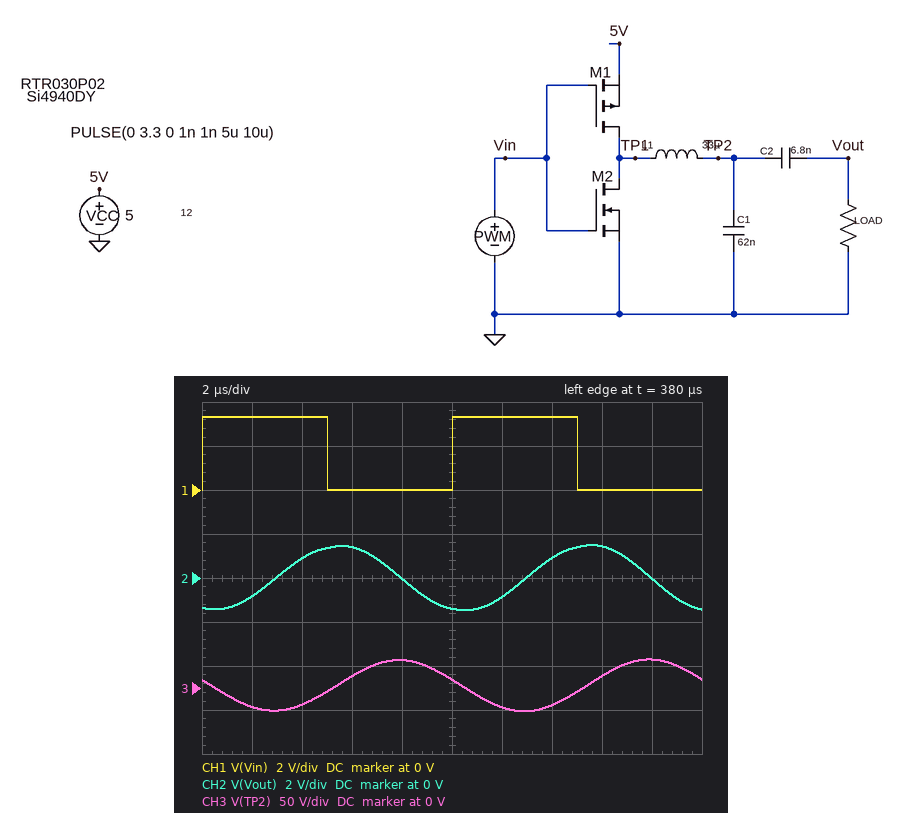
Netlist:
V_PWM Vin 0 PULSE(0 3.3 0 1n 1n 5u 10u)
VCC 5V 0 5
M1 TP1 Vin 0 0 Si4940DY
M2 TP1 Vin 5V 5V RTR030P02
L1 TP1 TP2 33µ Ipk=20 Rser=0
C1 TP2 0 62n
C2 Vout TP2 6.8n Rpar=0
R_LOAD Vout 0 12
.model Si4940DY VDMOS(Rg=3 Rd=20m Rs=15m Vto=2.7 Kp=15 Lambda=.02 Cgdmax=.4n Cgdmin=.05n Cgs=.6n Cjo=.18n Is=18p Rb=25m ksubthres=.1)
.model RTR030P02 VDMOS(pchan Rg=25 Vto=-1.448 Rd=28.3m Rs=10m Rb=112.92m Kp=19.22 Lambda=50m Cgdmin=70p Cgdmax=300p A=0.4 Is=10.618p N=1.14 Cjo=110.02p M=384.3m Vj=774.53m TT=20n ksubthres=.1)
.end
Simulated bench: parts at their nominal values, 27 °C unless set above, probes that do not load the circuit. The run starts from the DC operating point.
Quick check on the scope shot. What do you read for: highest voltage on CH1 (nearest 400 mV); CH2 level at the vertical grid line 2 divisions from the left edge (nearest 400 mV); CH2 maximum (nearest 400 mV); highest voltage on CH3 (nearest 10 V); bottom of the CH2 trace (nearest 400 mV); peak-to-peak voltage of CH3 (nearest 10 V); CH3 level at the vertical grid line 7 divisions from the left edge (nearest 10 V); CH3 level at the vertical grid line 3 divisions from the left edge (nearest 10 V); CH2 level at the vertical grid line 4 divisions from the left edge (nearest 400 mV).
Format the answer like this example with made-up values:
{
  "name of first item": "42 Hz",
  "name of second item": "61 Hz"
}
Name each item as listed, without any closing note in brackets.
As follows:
{
  "highest voltage on CH1": "3.2 V",
  "CH2 level at the vertical grid line 2 divisions from the left edge": "800 mV",
  "CH2 maximum": "1.6 V",
  "highest voltage on CH3": "30 V",
  "bottom of the CH2 trace": "-1.6 V",
  "peak-to-peak voltage of CH3": "60 V",
  "CH3 level at the vertical grid line 7 divisions from the left edge": "-20 V",
  "CH3 level at the vertical grid line 3 divisions from the left edge": "10 V",
  "CH2 level at the vertical grid line 4 divisions from the left edge": "0 V"
}
